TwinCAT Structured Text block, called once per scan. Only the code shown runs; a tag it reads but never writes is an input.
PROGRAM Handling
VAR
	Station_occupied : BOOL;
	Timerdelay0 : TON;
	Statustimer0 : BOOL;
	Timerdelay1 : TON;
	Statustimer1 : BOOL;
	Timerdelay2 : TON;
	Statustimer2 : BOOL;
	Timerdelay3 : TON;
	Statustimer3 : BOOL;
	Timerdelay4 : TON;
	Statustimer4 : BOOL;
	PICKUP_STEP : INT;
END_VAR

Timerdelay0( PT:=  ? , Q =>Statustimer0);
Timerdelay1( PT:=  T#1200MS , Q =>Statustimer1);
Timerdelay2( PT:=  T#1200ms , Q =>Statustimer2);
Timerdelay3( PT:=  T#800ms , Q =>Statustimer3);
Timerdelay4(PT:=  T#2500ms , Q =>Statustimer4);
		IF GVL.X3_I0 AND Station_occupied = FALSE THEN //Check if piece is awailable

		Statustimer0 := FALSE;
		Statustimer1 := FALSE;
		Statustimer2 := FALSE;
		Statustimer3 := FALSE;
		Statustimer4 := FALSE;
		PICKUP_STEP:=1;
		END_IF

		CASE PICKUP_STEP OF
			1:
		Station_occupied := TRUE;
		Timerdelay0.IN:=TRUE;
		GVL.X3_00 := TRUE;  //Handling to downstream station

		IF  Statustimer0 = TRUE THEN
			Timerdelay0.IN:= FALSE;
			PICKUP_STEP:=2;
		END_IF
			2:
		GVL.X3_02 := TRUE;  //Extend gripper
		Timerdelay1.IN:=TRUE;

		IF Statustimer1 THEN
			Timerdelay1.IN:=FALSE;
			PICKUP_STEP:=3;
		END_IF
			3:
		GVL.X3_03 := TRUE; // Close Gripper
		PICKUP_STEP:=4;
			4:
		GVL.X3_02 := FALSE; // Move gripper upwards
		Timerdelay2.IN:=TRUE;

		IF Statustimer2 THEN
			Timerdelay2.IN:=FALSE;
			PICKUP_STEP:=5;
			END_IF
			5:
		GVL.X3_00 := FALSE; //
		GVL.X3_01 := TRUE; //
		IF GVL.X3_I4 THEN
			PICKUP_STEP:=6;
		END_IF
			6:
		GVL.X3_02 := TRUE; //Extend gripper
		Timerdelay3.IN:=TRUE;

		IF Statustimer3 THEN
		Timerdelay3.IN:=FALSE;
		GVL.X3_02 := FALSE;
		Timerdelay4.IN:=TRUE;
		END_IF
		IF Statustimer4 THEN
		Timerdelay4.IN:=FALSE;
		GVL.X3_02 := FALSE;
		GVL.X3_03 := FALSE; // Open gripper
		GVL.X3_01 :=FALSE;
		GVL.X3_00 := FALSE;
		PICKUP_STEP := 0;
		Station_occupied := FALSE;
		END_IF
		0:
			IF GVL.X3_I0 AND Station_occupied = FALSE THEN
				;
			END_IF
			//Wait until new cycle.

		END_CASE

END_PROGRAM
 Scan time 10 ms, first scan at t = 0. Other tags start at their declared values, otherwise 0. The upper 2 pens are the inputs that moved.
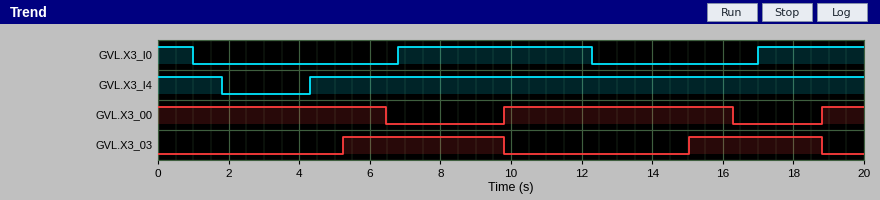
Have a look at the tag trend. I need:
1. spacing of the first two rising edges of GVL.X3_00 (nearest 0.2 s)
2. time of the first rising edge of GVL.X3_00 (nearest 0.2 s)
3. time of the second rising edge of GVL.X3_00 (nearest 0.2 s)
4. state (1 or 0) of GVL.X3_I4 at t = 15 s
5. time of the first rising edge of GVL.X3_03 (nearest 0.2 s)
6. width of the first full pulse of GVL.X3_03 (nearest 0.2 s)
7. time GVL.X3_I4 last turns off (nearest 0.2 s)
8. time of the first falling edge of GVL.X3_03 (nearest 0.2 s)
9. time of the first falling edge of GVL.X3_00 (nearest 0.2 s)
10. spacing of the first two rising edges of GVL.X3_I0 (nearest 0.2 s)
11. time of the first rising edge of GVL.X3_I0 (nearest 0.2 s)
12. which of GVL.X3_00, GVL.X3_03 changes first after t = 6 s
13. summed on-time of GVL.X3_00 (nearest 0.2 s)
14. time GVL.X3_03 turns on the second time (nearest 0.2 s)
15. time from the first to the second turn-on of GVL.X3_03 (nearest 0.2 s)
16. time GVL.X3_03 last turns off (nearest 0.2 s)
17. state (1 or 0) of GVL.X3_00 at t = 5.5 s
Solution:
9.0 s
9.8 s
18.8 s
1
5.2 s
4.6 s
1.8 s
9.8 s
6.4 s
10.2 s
6.8 s
GVL.X3_00
14.2 s
15.0 s
9.8 s
18.8 s
1
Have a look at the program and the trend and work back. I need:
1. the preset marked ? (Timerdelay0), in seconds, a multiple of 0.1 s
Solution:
4.0 s
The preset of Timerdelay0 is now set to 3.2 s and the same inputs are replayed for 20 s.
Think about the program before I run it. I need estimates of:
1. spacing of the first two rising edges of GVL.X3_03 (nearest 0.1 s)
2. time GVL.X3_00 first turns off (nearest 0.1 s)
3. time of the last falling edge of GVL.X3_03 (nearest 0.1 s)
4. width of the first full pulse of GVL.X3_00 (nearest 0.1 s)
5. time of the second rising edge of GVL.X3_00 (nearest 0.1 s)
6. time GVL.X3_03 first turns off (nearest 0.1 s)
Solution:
9.0 s
5.7 s
17.2 s
5.7 s
17.2 s
9.0 s
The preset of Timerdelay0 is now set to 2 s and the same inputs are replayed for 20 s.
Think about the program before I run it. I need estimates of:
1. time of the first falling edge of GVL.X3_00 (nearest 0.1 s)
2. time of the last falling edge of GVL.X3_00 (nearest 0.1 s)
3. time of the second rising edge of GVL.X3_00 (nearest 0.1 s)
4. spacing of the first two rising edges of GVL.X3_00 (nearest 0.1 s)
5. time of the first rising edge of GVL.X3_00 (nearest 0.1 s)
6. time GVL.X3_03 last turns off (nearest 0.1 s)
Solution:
4.5 s
12.3 s
17.0 s
9.2 s
7.8 s
14.8 s
